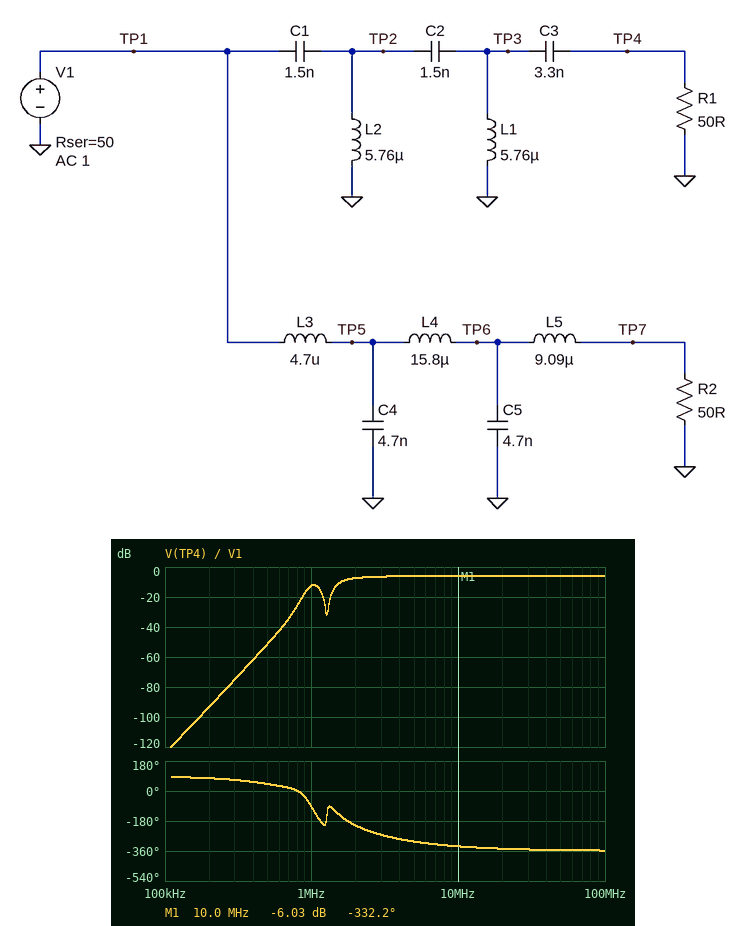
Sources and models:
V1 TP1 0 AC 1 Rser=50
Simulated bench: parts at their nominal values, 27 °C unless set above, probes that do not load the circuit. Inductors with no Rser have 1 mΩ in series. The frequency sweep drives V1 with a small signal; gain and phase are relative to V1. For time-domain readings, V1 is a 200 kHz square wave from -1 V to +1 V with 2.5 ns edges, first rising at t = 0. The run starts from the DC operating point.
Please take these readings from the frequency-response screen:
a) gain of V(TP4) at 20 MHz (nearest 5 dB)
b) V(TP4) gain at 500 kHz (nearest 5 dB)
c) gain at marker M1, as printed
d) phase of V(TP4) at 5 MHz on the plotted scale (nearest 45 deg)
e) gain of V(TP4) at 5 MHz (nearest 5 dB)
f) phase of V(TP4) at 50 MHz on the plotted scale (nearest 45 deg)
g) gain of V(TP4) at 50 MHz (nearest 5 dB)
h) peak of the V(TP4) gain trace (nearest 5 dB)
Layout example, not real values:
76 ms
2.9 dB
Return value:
-5 dB
-50 dB
-6.03 dB
-315 deg
-5 dB
-360 deg
-5 dB
-5 dB
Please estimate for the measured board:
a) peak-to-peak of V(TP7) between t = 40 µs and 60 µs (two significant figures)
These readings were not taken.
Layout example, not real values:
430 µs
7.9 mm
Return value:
1.2 V
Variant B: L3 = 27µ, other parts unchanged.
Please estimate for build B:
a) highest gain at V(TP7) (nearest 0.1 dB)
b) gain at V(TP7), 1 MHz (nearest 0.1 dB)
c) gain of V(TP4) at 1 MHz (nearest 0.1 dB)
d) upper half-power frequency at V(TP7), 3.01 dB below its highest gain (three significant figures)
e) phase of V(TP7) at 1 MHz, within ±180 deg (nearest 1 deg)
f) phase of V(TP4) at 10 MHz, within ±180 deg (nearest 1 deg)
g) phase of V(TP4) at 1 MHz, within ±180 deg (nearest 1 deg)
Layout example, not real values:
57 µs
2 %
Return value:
-6.0 dB
-14.1 dB
-7.5 dB
811 kHz
12 deg
24 deg
-72 deg
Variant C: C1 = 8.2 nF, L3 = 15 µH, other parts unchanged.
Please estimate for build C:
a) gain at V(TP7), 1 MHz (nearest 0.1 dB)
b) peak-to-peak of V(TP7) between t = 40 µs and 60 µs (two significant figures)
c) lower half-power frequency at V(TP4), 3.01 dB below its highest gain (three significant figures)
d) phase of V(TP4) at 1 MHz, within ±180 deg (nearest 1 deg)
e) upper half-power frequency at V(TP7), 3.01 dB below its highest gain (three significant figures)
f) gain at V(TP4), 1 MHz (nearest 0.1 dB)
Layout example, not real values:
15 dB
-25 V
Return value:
-10.4 dB
1.3 V
1.12 MHz
-140 deg
457 kHz
-12.6 dB
